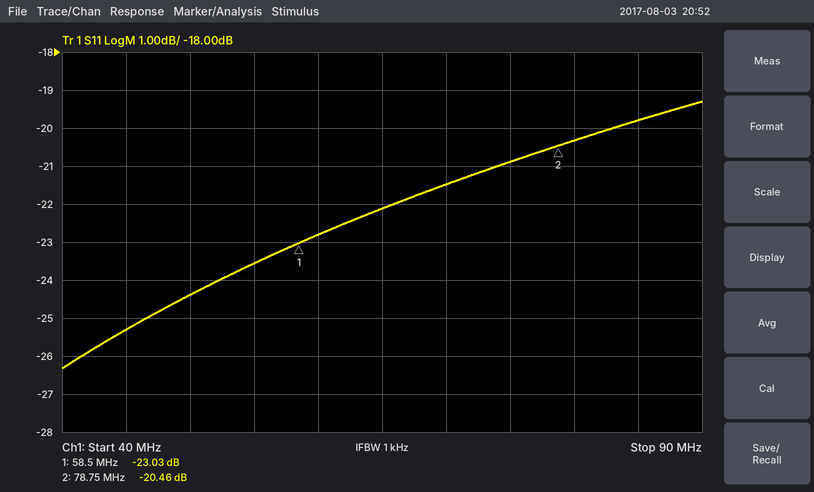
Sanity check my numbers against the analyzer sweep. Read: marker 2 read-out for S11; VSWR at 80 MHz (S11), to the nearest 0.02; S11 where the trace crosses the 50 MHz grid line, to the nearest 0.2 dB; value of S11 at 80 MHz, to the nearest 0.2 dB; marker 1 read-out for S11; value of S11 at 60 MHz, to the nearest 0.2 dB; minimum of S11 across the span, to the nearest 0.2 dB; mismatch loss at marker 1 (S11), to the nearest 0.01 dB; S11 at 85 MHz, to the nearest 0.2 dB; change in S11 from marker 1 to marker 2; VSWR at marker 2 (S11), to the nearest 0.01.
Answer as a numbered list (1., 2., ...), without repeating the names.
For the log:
1. -20.46 dB
2. 1.22
3. -24.4 dB
4. -20.4 dB
5. -23.03 dB
6. -22.8 dB
7. -26.4 dB
8. 0.02 dB
9. -19.8 dB
10. 2.57 dB
11. 1.21
